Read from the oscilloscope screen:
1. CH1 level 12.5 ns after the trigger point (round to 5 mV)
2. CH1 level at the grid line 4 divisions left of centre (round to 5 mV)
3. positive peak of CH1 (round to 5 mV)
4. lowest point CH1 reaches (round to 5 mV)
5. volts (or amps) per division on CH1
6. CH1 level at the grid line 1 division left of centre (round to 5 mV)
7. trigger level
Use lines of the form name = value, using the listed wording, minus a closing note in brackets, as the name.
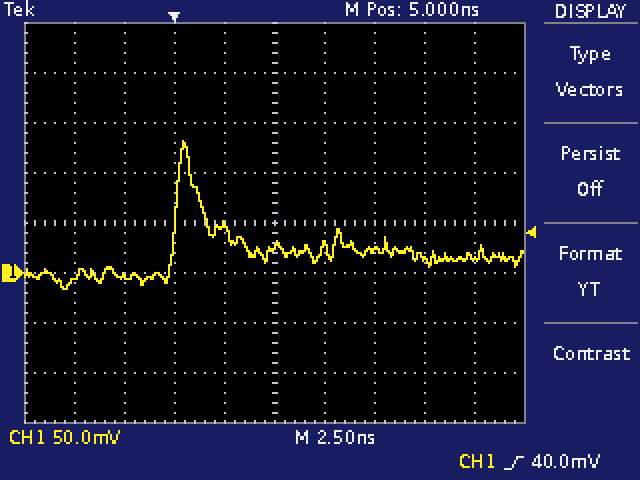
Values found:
CH1 level 12.5 ns after the trigger point = 15 mV
CH1 level at the grid line 4 divisions left of centre = -5 mV
positive peak of CH1 = 130 mV
lowest point CH1 reaches = -15 mV
volts (or amps) per division on CH1 = 50 mV
CH1 level at the grid line 1 division left of centre = 45 mV
trigger level = 40.0 mV
